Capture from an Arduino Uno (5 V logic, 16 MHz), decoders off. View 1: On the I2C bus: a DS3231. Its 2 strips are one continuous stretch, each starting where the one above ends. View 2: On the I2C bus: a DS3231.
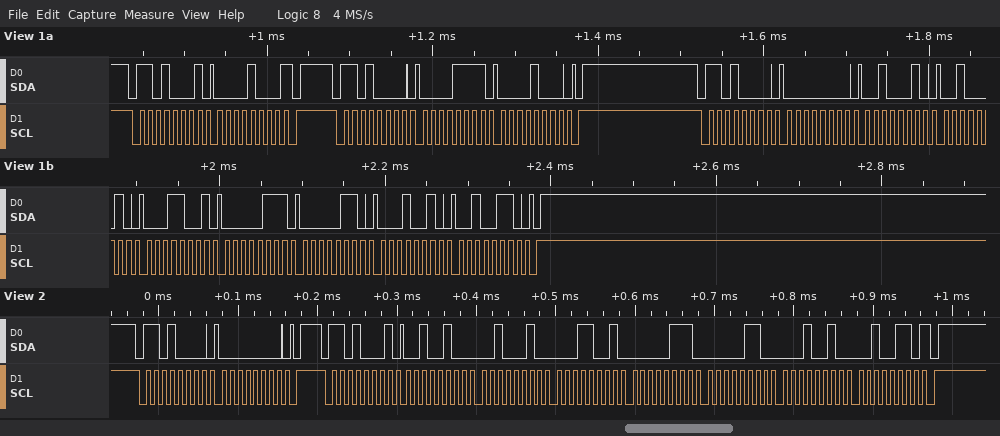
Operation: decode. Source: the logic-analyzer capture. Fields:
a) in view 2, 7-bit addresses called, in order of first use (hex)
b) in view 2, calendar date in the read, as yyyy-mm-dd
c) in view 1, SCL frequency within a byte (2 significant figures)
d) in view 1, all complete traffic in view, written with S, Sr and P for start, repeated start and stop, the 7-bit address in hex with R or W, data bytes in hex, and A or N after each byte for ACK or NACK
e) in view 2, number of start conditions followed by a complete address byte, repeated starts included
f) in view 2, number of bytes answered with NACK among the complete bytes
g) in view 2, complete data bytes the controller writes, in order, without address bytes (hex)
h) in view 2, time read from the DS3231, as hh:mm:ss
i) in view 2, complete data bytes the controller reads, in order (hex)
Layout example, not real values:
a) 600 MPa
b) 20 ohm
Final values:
a) 0x68
b) 2026-12-06
c) 100 kHz
d) S 68R A 08 N P S 68W A 0F A 08 A P S 68W A 00 A 22 A 22 A 19 A 07 A 06 A 12 A 26 A P
e) 2
f) 1
g) 00
h) 19:22:24
i) 24 22 19 07 06 12 26
